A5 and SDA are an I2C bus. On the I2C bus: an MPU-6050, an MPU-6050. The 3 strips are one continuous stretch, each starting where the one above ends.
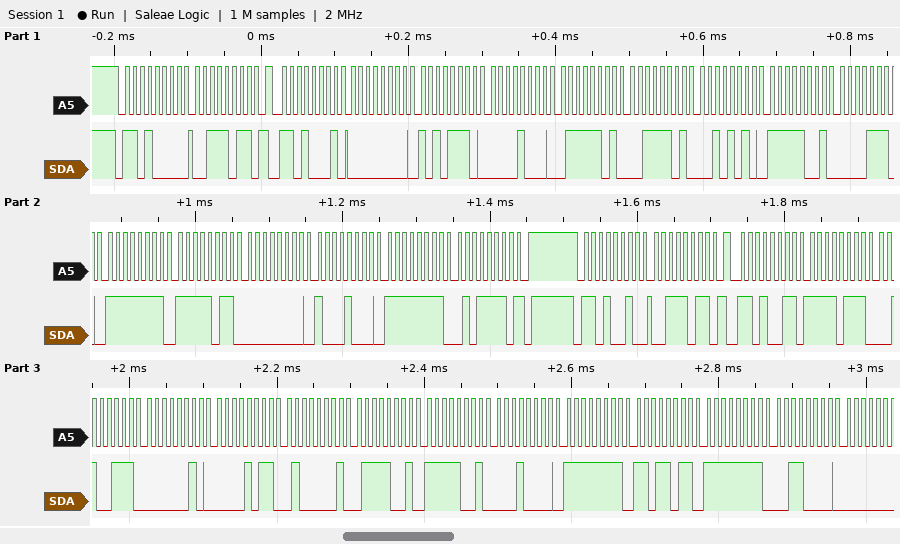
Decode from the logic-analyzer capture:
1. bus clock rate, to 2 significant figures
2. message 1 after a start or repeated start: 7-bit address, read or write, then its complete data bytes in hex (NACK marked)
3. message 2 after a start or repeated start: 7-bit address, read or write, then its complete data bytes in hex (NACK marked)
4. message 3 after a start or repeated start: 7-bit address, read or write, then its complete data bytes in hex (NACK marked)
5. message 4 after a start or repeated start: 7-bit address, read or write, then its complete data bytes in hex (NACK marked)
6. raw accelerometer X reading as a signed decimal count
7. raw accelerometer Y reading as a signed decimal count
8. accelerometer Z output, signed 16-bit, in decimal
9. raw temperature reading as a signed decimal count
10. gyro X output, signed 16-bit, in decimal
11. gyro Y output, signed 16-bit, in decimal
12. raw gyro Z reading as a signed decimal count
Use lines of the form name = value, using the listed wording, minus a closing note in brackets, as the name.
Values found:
bus clock rate, to 2 significant figures = 100 kHz
message 1 after a start or repeated start: 7-bit address, read or write, then its complete data bytes in hex = 0x68 write: 3B
message 2 after a start or repeated start: 7-bit address, read or write, then its complete data bytes in hex = 0x68 read: 00 AE 08 7D 3D 2A F9 0E FF FB 00 88 FF 5E NACK
message 3 after a start or repeated start: 7-bit address, read or write, then its complete data bytes in hex = 0x69 write: 3B
message 4 after a start or repeated start: 7-bit address, read or write, then its complete data bytes in hex = 0x69 read: F7 27 02 0B 41 79 F9 10 FF DB FF 30
raw accelerometer X reading as a signed decimal count = 174
raw accelerometer Y reading as a signed decimal count = 2173
accelerometer Z output, signed 16-bit, in decimal = 15658
raw temperature reading as a signed decimal count = -1778
gyro X output, signed 16-bit, in decimal = -5
gyro Y output, signed 16-bit, in decimal = 136
raw gyro Z reading as a signed decimal count = -162
